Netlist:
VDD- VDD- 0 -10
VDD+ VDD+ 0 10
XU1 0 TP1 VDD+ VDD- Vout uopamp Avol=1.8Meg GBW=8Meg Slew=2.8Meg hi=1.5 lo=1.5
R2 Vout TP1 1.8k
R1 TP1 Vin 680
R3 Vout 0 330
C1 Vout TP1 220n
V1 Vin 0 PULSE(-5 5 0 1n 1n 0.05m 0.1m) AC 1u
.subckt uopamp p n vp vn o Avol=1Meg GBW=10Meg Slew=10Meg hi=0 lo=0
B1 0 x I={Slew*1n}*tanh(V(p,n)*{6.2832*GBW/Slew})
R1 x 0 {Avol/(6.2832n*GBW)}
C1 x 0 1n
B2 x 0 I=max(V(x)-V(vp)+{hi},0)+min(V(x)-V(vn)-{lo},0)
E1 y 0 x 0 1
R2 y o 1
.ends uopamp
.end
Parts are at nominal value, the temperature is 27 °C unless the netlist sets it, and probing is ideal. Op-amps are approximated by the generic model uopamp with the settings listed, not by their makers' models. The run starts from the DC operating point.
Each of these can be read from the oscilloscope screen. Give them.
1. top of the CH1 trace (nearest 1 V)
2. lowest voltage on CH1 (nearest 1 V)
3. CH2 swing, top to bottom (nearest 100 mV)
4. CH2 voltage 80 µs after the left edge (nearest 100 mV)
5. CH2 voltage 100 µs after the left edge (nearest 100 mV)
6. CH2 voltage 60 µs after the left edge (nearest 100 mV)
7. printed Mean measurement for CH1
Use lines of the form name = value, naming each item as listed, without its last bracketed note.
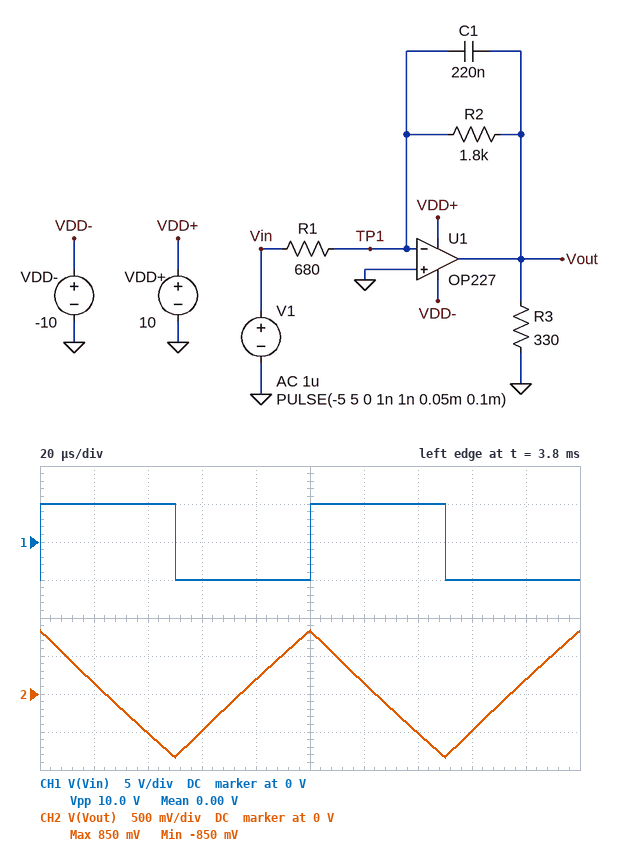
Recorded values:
top of the CH1 trace = 5 V
lowest voltage on CH1 = -5 V
CH2 swing, top to bottom = 1.7 V
CH2 voltage 80 µs after the left edge = 200 mV
CH2 voltage 100 µs after the left edge = 800 mV
CH2 voltage 60 µs after the left edge = -500 mV
printed Mean measurement for CH1 = 0.00 V
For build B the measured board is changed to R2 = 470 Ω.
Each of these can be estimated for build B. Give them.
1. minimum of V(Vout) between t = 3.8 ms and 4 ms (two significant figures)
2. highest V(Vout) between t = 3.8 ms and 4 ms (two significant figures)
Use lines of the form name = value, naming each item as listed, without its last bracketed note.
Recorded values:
minimum of V(Vout) between t = 3.8 ms and 4 ms = -830 mV
highest V(Vout) between t = 3.8 ms and 4 ms = 830 mV
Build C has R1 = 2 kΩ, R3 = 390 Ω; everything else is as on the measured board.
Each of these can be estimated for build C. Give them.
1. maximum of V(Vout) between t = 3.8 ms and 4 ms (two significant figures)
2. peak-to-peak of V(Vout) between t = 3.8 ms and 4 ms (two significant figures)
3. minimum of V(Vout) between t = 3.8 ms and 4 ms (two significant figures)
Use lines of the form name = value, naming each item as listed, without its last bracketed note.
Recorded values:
maximum of V(Vout) between t = 3.8 ms and 4 ms = 290 mV
peak-to-peak of V(Vout) between t = 3.8 ms and 4 ms = 580 mV
minimum of V(Vout) between t = 3.8 ms and 4 ms = -290 mV
